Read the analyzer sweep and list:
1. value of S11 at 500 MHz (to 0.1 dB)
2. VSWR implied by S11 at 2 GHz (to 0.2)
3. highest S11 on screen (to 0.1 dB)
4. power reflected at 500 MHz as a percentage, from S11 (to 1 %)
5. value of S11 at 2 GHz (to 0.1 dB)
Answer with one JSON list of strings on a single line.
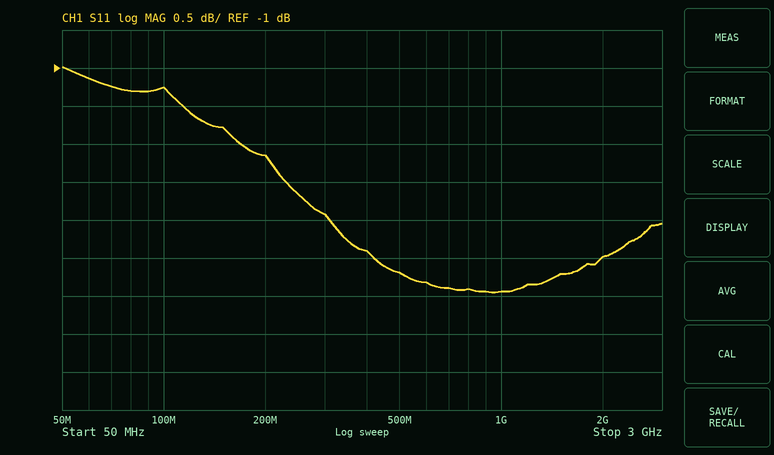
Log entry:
["-3.7 dB", "5.0", "-1.0 dB", "43 %", "-3.5 dB"]
